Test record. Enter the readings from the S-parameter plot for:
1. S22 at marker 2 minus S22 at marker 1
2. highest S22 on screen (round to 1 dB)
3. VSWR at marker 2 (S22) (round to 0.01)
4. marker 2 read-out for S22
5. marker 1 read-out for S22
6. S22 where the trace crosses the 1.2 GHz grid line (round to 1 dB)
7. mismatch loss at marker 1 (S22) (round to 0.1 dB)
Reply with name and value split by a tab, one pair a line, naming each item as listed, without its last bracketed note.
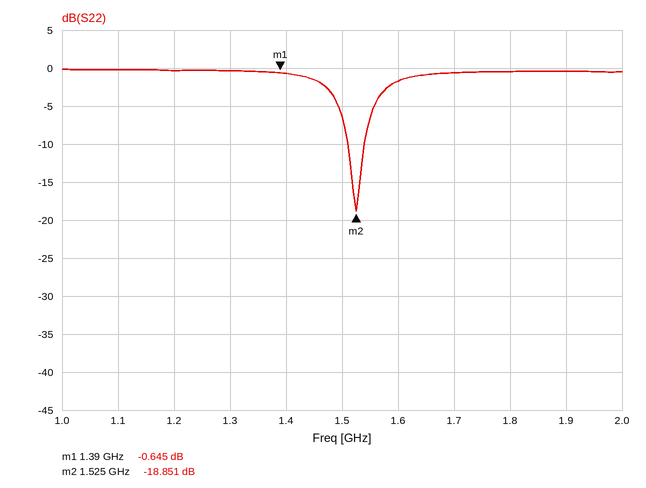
S22 at marker 2 minus S22 at marker 1	-18.206 dB
highest S22 on screen	0 dB
VSWR at marker 2 (S22)	1.26
marker 2 read-out for S22	-18.851 dB
marker 1 read-out for S22	-0.645 dB
S22 where the trace crosses the 1.2 GHz grid line	0 dB
mismatch loss at marker 1 (S22)	8.6 dB
